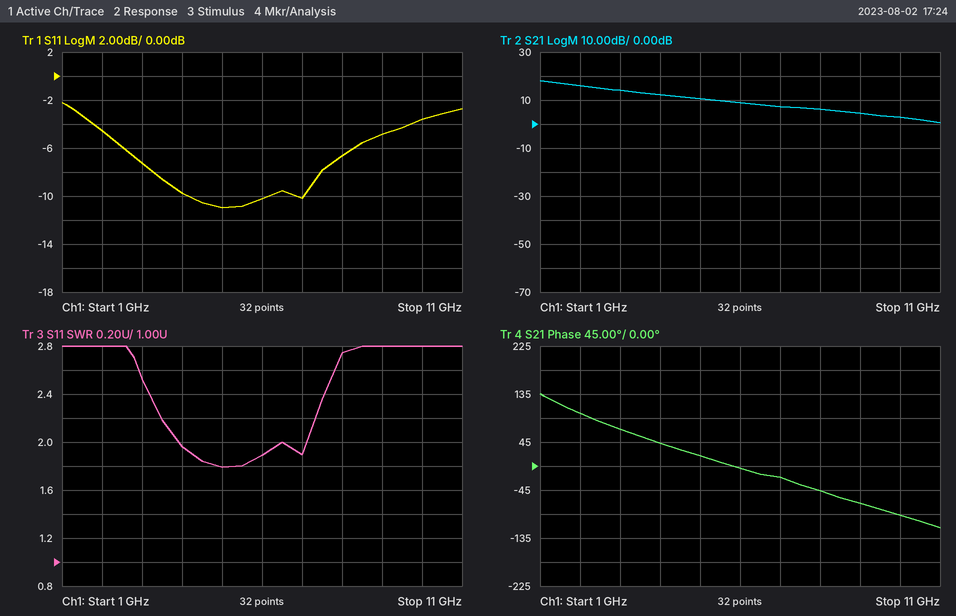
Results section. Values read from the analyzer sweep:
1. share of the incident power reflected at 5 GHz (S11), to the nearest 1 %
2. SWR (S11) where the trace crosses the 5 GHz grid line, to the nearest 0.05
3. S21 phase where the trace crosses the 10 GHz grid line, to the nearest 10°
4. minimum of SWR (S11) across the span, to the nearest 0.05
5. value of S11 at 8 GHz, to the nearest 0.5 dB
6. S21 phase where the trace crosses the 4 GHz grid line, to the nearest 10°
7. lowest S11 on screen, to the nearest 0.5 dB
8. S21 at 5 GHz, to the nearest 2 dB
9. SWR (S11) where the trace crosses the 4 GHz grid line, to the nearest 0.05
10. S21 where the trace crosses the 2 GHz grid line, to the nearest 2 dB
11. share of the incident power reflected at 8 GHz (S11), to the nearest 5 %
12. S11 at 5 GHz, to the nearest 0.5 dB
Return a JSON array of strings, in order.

["8 %", "1.80", "-90°", "1.80", "-6.5 dB", "40°", "-11.0 dB", "10 dB", "1.95", "16 dB", "20 %", "-11.0 dB"]
